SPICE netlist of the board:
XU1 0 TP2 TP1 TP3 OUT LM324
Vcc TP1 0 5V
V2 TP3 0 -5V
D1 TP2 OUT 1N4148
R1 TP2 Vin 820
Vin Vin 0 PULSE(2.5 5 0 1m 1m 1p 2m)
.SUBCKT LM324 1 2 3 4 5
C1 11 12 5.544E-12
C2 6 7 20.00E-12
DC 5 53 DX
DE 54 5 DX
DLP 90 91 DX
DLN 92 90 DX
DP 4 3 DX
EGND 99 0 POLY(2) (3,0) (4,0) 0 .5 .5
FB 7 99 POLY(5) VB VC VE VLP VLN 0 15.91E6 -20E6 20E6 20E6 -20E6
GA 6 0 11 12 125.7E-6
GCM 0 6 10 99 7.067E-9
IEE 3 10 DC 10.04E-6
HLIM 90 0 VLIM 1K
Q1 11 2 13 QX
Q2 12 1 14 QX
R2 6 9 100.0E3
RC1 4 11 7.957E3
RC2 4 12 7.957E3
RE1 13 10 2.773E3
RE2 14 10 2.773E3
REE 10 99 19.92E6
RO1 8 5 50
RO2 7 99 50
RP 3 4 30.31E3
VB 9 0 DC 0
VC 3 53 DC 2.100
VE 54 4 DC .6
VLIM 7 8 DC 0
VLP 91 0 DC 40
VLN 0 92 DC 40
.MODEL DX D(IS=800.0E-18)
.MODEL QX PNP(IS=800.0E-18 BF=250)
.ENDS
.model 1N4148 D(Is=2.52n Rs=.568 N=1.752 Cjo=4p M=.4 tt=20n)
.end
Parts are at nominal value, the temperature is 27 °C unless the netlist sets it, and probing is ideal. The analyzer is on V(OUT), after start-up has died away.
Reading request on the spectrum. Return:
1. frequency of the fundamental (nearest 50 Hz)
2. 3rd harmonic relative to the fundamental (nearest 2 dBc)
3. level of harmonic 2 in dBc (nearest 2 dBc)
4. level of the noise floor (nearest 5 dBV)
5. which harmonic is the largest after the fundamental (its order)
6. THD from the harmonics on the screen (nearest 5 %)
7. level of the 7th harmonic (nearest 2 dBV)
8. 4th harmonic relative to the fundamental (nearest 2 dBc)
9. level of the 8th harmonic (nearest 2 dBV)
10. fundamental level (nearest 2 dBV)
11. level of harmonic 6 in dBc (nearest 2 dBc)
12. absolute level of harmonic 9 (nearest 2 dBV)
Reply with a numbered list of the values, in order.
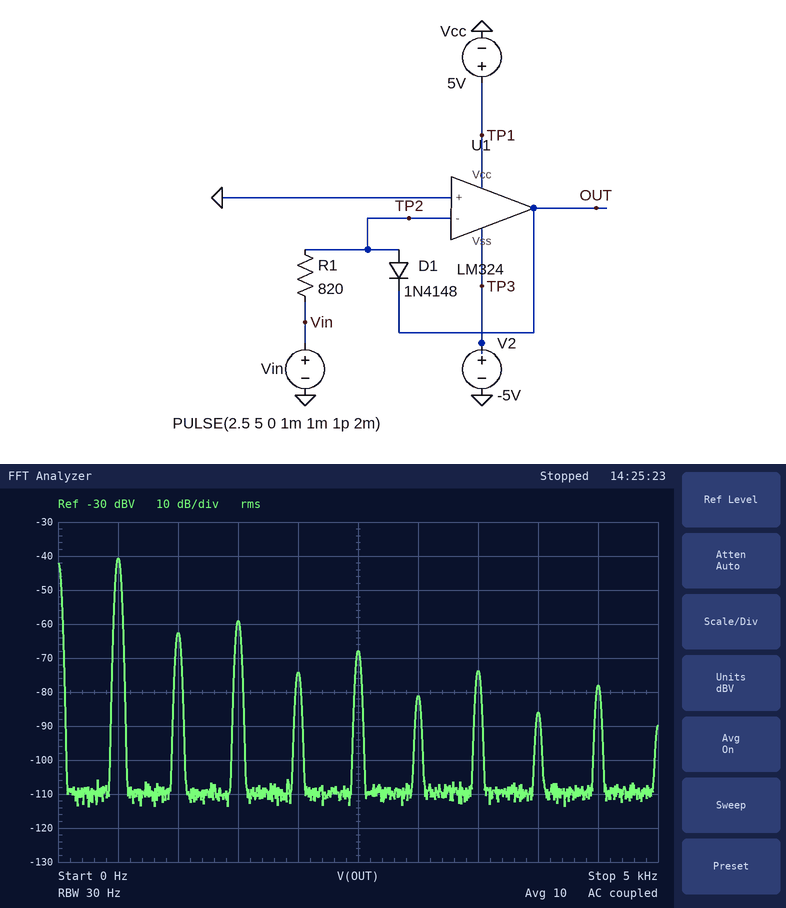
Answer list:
1. 500 Hz
2. -18 dBc
3. -22 dBc
4. -110 dBV
5. 3
6. 15 %
7. -74 dBV
8. -34 dBc
9. -86 dBV
10. -40 dBV
11. -40 dBc
12. -78 dBV
